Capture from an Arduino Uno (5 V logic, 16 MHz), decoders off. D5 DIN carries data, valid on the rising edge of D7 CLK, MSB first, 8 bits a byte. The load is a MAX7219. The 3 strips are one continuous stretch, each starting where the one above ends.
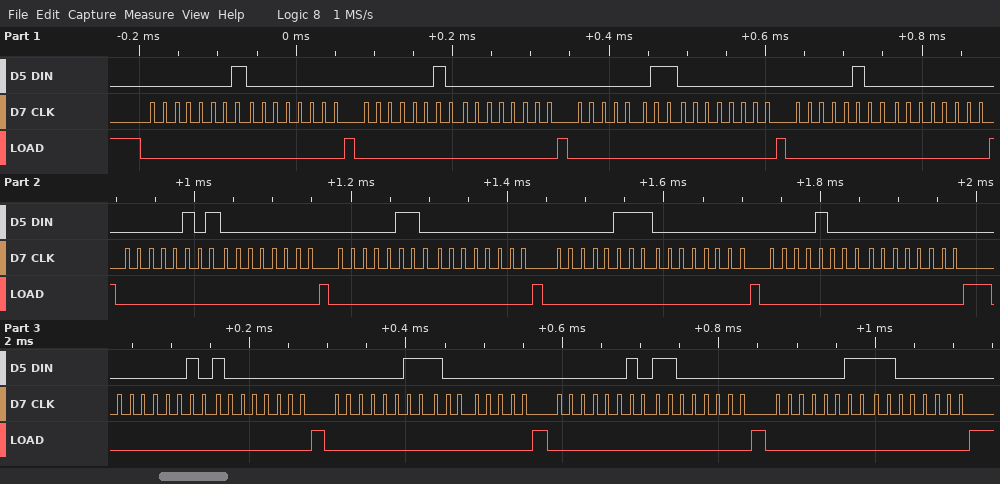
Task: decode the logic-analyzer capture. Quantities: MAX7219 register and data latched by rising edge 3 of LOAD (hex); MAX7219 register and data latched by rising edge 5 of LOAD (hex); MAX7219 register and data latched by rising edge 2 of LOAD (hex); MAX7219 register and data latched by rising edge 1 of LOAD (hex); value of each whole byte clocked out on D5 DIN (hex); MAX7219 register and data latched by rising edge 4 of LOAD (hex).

register 0x3, data 0x00
register 0x5, data 0x00
register 0x2, data 0x00
register 0x1, data 0x00
0x01 0x00 0x02 0x00 0x03 0x00 0x04 0x00 0x05 0x00 0x06 0x00 0x07 0x00 0x08 0x00 0x02 0x80 0x03 0x80 0x02 0xC0 0x03 0xC0
register 0x4, data 0x00
